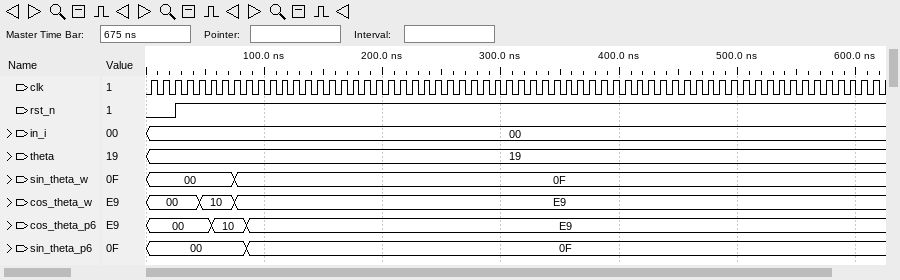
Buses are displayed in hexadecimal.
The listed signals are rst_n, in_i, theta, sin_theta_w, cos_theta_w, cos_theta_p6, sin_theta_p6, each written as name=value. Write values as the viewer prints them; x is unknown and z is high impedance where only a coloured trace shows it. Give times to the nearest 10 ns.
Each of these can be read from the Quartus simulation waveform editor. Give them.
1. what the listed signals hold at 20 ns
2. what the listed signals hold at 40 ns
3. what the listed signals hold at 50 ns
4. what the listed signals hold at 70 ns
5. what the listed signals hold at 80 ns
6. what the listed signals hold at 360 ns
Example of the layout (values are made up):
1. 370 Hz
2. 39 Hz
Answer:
1. rst_n=0, in_i=00, theta=19, sin_theta_w=00, cos_theta_w=00, cos_theta_p6=00, sin_theta_p6=00
2. rst_n=1, in_i=00, theta=19, sin_theta_w=00, cos_theta_w=00, cos_theta_p6=00, sin_theta_p6=00
3. rst_n=1, in_i=00, theta=19, sin_theta_w=00, cos_theta_w=10, cos_theta_p6=00, sin_theta_p6=00
4. rst_n=1, in_i=00, theta=19, sin_theta_w=00, cos_theta_w=10, cos_theta_p6=10, sin_theta_p6=00
5. rst_n=1, in_i=00, theta=19, sin_theta_w=0F, cos_theta_w=E9, cos_theta_p6=10, sin_theta_p6=00
6. rst_n=1, in_i=00, theta=19, sin_theta_w=0F, cos_theta_w=E9, cos_theta_p6=E9, sin_theta_p6=0F
